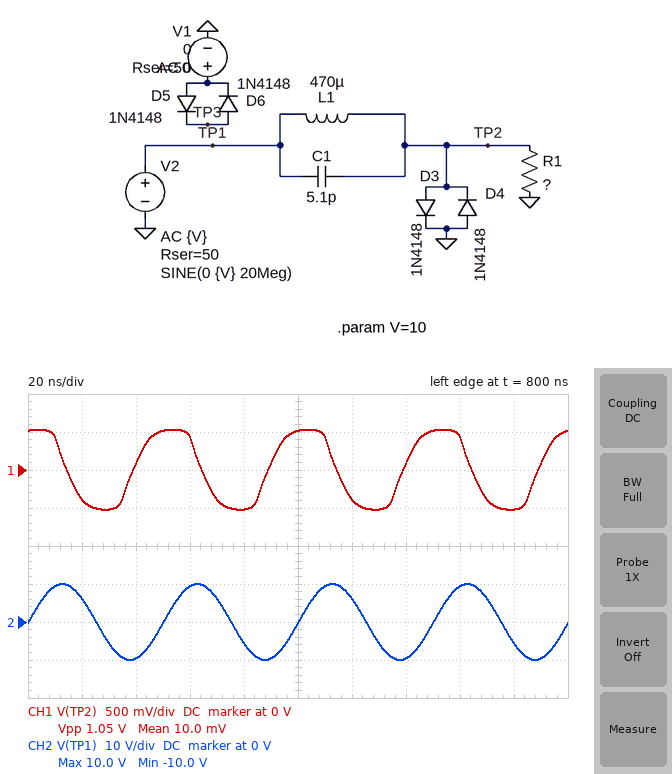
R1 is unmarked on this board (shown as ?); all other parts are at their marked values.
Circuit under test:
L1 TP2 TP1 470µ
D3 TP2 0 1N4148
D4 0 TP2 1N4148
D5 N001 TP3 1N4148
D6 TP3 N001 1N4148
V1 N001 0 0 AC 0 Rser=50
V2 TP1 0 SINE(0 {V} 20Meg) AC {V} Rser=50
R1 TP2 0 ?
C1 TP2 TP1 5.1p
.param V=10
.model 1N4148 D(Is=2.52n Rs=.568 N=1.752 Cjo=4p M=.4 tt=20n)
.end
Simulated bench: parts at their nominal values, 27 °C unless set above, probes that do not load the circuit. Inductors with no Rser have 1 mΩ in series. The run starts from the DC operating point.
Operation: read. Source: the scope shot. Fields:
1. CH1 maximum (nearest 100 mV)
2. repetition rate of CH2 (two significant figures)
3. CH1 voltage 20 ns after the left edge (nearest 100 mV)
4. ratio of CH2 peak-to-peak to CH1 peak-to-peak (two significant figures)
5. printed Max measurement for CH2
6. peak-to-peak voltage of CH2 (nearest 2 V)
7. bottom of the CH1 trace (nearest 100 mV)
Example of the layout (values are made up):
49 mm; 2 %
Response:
500 mV; 20 MHz; -400 mV; 19; 10.0 V; 20 V; -500 mV
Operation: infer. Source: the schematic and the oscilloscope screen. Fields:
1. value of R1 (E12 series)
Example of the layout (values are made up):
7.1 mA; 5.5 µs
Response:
100 Ω
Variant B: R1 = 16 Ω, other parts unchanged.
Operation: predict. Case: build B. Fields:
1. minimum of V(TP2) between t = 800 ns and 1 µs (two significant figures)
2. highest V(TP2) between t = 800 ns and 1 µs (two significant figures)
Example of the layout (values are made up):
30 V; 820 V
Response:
-97 mV; 100 mV
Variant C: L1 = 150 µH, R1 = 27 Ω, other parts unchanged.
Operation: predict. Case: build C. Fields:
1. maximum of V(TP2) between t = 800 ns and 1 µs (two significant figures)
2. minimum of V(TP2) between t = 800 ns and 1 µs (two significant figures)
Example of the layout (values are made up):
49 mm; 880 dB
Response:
170 mV; -150 mV
